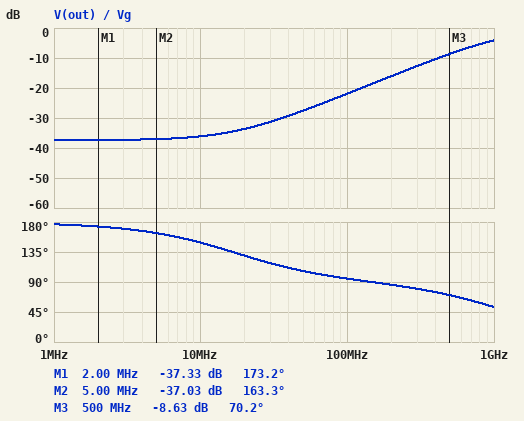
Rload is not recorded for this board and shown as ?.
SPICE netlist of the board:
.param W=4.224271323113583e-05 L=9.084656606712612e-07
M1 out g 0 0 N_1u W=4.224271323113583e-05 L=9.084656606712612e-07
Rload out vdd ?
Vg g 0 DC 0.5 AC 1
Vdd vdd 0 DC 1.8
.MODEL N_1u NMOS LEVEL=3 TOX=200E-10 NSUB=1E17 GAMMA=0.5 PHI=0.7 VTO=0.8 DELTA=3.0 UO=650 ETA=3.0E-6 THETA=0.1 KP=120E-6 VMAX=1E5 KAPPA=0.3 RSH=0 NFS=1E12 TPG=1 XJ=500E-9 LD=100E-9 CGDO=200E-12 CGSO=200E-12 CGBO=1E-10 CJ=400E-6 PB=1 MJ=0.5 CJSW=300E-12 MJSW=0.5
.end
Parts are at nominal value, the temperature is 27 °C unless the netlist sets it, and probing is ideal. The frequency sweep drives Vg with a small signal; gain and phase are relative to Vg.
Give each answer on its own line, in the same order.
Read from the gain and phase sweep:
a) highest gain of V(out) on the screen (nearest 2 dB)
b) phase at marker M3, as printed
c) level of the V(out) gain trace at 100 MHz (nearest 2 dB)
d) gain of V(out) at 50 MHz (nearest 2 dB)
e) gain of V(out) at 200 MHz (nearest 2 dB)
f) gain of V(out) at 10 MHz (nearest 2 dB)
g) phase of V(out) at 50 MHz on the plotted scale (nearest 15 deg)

-4 dB
70.2 deg
-22 dB
-28 dB
-16 dB
-36 dB
105 deg
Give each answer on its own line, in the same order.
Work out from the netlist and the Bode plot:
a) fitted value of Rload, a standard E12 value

15 kΩ
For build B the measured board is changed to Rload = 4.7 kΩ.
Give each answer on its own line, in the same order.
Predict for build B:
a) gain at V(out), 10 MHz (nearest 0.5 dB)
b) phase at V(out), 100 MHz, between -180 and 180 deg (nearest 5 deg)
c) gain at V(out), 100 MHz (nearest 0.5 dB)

-46.0 dB
100 deg
-32.0 dB
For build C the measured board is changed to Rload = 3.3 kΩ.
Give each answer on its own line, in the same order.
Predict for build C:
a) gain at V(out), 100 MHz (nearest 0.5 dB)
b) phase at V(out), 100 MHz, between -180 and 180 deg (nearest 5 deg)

-35.0 dB
100 deg
